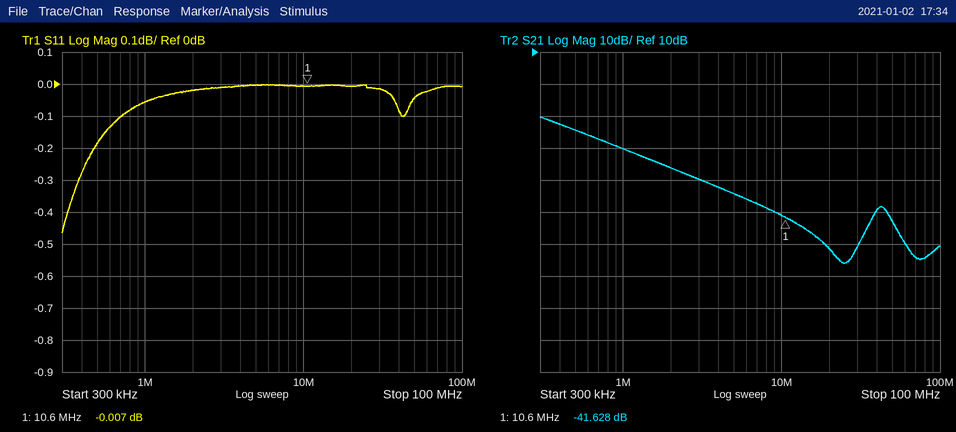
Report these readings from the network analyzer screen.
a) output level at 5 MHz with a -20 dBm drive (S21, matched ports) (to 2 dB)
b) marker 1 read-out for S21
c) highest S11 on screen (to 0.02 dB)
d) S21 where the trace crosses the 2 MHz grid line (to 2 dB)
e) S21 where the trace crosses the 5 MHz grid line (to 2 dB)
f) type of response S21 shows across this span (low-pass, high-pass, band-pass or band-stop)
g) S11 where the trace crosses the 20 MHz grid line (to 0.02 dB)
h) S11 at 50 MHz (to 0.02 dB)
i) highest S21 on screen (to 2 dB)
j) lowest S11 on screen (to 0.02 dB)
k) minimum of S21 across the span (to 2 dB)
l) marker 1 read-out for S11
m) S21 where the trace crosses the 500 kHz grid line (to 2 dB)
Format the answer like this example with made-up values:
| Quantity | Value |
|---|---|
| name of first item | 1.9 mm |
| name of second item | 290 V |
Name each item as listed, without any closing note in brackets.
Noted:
| Quantity | Value |
|---|---|
| output level at 5 MHz with a -20 dBm drive (S21, matched ports) | -54 dBm |
| marker 1 read-out for S21 | -41.628 dB |
| highest S11 on screen | 0.00 dB |
| S21 where the trace crosses the 2 MHz grid line | -26 dB |
| S21 where the trace crosses the 5 MHz grid line | -34 dB |
| type of response S21 shows across this span | low-pass |
| S11 where the trace crosses the 20 MHz grid line | 0.00 dB |
| S11 at 50 MHz | -0.04 dB |
| highest S21 on screen | -10 dB |
| lowest S11 on screen | -0.46 dB |
| minimum of S21 across the span | -56 dB |
| marker 1 read-out for S11 | -0.007 dB |
| S21 where the trace crosses the 500 kHz grid line | -14 dB |
